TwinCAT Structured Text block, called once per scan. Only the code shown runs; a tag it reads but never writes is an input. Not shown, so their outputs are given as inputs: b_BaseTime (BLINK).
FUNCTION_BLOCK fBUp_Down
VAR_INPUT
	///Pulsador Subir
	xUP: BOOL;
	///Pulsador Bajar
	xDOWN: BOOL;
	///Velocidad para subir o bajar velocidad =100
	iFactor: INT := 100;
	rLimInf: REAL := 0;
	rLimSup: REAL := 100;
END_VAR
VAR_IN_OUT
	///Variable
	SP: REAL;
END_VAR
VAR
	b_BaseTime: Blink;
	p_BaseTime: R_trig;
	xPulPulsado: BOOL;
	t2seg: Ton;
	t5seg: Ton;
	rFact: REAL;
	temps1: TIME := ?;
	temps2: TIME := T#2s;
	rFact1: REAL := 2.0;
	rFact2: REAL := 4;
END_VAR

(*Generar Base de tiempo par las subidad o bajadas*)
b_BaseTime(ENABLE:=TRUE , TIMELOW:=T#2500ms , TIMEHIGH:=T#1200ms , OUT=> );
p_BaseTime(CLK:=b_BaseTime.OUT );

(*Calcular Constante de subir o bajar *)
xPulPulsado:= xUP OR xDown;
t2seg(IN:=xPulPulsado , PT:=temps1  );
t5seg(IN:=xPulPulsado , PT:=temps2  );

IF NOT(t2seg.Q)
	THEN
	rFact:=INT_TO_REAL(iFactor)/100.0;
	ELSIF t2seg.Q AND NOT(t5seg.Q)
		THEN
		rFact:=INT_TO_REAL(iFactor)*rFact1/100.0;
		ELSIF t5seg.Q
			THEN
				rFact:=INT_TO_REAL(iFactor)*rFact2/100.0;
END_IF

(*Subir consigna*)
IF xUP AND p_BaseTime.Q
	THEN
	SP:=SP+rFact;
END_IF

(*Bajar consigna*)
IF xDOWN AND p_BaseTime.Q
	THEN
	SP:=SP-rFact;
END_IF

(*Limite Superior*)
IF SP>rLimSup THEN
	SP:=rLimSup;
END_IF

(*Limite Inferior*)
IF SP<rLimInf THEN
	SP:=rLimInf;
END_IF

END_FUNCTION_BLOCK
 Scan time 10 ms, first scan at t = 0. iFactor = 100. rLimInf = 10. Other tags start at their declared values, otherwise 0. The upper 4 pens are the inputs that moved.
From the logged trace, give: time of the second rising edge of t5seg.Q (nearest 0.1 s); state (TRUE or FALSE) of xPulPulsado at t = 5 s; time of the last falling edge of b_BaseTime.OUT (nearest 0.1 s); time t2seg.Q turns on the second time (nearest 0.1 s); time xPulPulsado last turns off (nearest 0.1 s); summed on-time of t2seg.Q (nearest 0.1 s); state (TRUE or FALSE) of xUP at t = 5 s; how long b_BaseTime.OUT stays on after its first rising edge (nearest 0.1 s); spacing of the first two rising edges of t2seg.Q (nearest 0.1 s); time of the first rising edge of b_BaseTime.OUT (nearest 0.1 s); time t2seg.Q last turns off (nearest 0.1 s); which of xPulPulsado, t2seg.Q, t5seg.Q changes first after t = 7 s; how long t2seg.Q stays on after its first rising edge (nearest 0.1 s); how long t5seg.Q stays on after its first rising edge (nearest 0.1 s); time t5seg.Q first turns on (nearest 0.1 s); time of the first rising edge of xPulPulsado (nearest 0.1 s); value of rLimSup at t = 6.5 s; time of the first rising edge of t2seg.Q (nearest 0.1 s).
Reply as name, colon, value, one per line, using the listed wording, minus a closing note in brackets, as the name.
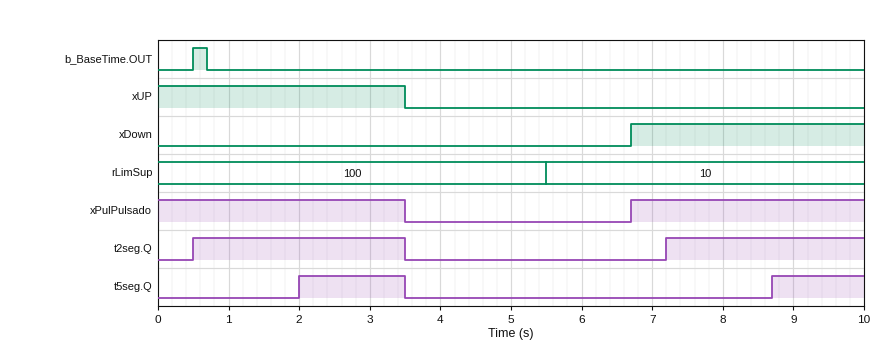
time of the second rising edge of t5seg.Q: 8.7 s
state (TRUE or FALSE) of xPulPulsado at t = 5 s: FALSE
time of the last falling edge of b_BaseTime.OUT: 0.7 s
time t2seg.Q turns on the second time: 7.2 s
time xPulPulsado last turns off: 3.5 s
summed on-time of t2seg.Q: 5.8 s
state (TRUE or FALSE) of xUP at t = 5 s: FALSE
how long b_BaseTime.OUT stays on after its first rising edge: 0.2 s
spacing of the first two rising edges of t2seg.Q: 6.7 s
time of the first rising edge of b_BaseTime.OUT: 0.5 s
time t2seg.Q last turns off: 3.5 s
which of xPulPulsado, t2seg.Q, t5seg.Q changes first after t = 7 s: t2seg.Q
how long t2seg.Q stays on after its first rising edge: 3.0 s
how long t5seg.Q stays on after its first rising edge: 1.5 s
time t5seg.Q first turns on: 2.0 s
time of the first rising edge of xPulPulsado: 6.7 s
value of rLimSup at t = 6.5 s: 10
time of the first rising edge of t2seg.Q: 0.5 s
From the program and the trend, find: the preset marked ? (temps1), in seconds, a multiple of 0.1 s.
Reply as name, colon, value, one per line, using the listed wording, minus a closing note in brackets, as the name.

the preset marked ? (temps1), in seconds, a multiple of 0.1 s: 0.5 s
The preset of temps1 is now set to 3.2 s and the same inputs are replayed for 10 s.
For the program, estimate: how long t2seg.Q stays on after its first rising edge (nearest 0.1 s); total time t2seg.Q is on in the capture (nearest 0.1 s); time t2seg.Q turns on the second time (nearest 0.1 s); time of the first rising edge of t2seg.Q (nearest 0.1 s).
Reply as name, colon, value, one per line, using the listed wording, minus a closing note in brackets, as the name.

how long t2seg.Q stays on after its first rising edge: 0.3 s
total time t2seg.Q is on in the capture: 0.4 s
time t2seg.Q turns on the second time: 9.9 s
time of the first rising edge of t2seg.Q: 3.2 s
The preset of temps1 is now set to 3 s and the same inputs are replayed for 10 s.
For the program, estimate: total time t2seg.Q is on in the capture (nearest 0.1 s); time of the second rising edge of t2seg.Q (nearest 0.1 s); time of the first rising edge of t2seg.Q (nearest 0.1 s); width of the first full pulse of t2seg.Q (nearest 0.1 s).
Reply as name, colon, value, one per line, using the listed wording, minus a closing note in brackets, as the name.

total time t2seg.Q is on in the capture: 0.8 s
time of the second rising edge of t2seg.Q: 9.7 s
time of the first rising edge of t2seg.Q: 3.0 s
width of the first full pulse of t2seg.Q: 0.5 s
